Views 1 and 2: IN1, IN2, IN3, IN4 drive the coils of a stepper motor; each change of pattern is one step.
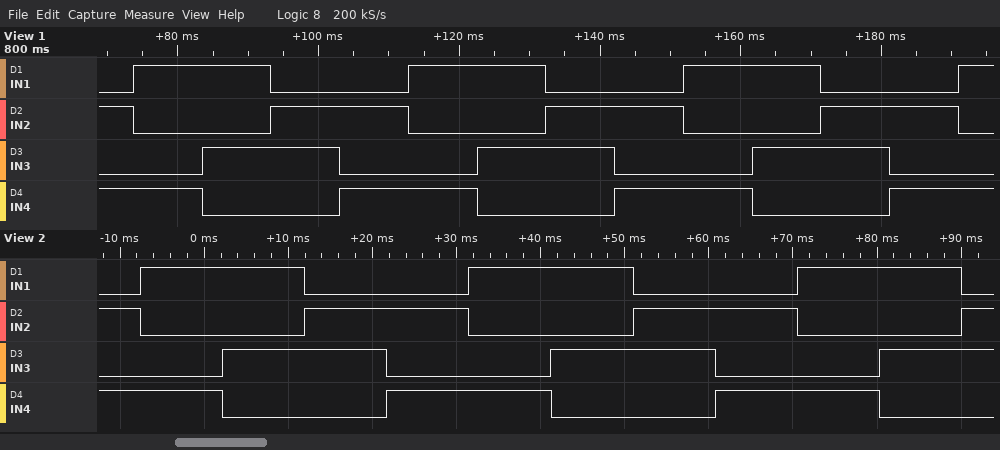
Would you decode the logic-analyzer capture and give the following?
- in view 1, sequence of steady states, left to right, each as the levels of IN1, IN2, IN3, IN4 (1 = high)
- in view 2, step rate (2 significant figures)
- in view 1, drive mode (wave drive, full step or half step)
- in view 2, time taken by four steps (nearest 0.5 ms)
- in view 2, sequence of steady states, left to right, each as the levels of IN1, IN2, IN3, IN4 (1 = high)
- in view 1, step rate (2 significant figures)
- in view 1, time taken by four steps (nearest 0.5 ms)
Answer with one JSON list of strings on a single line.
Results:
["0101 1001 1010 0110 0101 1001 1010 0110 0101 1001 1010 0110 0101 1001", "100 steps/s", "full step", "39.0 ms", "0101 1001 1010 0110 0101 1001 1010 0110 0101 1001 1010 0110", "100 steps/s", "39.0 ms"]
